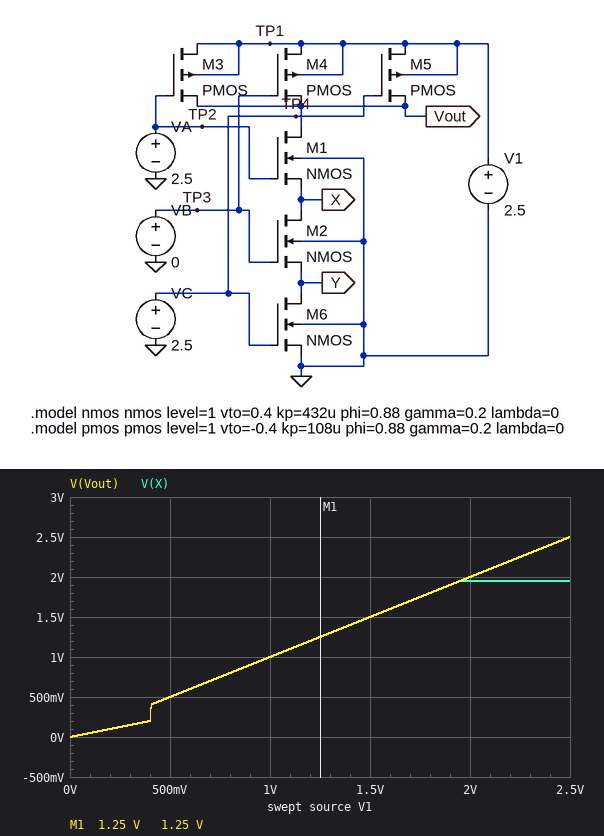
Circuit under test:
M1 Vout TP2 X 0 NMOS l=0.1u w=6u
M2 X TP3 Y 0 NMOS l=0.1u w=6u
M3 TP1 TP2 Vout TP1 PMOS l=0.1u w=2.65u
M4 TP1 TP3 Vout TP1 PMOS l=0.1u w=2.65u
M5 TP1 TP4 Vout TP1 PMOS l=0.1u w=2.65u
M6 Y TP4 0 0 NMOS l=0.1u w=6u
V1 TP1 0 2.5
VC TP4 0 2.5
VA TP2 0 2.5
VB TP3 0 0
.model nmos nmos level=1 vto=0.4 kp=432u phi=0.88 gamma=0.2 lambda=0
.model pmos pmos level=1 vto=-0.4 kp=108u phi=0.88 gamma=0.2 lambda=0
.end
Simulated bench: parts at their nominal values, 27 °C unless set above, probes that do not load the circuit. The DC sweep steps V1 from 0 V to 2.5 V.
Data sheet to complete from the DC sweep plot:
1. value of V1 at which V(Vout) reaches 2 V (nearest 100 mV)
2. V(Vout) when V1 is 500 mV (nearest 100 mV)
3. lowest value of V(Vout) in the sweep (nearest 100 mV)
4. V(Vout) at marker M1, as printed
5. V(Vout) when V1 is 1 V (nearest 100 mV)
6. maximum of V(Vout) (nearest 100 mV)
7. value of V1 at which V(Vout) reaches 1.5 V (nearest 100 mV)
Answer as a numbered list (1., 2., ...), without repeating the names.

1. 2.0 V
2. 500 mV
3. 0 V
4. 1.25 V
5. 1.0 V
6. 2.5 V
7. 1.5 V
